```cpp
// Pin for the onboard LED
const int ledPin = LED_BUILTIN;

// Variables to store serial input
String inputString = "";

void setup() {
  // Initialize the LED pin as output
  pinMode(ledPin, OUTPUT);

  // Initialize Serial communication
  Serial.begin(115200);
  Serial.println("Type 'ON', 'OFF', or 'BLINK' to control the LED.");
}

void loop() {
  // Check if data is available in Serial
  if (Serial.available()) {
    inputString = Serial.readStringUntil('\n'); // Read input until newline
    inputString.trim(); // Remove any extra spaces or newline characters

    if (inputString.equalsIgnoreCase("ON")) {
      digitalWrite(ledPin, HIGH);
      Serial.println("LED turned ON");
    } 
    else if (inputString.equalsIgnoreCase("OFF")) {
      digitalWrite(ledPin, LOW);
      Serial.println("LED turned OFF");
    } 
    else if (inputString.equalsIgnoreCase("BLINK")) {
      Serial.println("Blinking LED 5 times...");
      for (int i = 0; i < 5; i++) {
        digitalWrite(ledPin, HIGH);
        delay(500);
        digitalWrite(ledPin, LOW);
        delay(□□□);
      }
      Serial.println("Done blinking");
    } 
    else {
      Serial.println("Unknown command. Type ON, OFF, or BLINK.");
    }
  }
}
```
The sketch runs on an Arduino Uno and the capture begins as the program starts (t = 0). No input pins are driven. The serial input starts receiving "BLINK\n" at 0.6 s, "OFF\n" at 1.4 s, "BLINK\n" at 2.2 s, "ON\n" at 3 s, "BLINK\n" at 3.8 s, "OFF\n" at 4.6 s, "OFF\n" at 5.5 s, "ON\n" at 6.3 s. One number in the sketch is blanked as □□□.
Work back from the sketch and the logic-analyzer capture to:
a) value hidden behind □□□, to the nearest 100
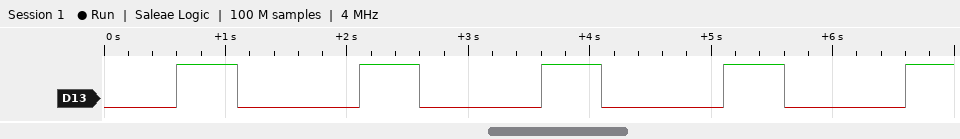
1000
